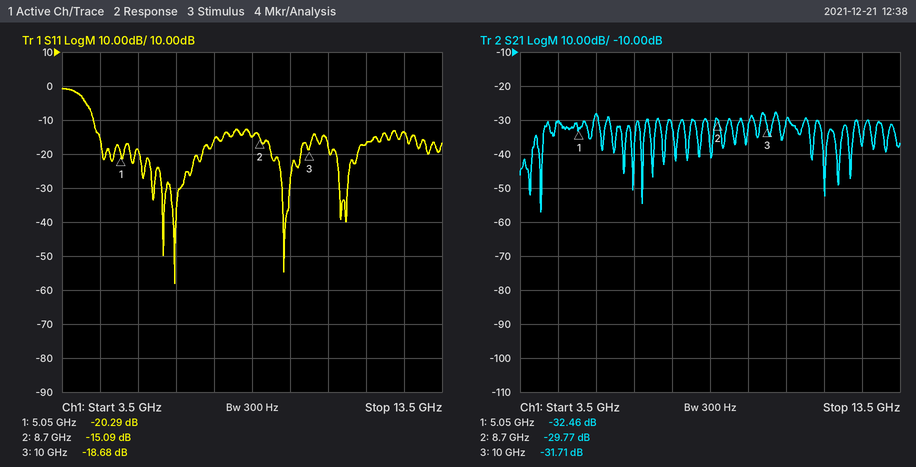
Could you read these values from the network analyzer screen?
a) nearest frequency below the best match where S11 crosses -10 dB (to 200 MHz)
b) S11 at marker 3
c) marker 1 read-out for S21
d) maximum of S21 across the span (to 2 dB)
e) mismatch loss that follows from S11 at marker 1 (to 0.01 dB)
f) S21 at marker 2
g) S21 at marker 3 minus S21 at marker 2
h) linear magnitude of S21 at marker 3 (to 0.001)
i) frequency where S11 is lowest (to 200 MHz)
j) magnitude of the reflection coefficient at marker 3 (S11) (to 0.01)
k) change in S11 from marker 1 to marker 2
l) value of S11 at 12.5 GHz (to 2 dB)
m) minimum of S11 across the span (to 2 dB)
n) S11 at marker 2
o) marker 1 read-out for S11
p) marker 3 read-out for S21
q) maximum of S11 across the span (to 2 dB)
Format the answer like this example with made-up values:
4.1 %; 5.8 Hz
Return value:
4.4 GHz; -18.68 dB; -32.46 dB; -28 dB; 0.04 dB; -29.77 dB; -1.94 dB; 0.026; 6.4 GHz; 0.12; 5.20 dB; -14 dB; -58 dB; -15.09 dB; -20.29 dB; -31.71 dB; 0 dB
